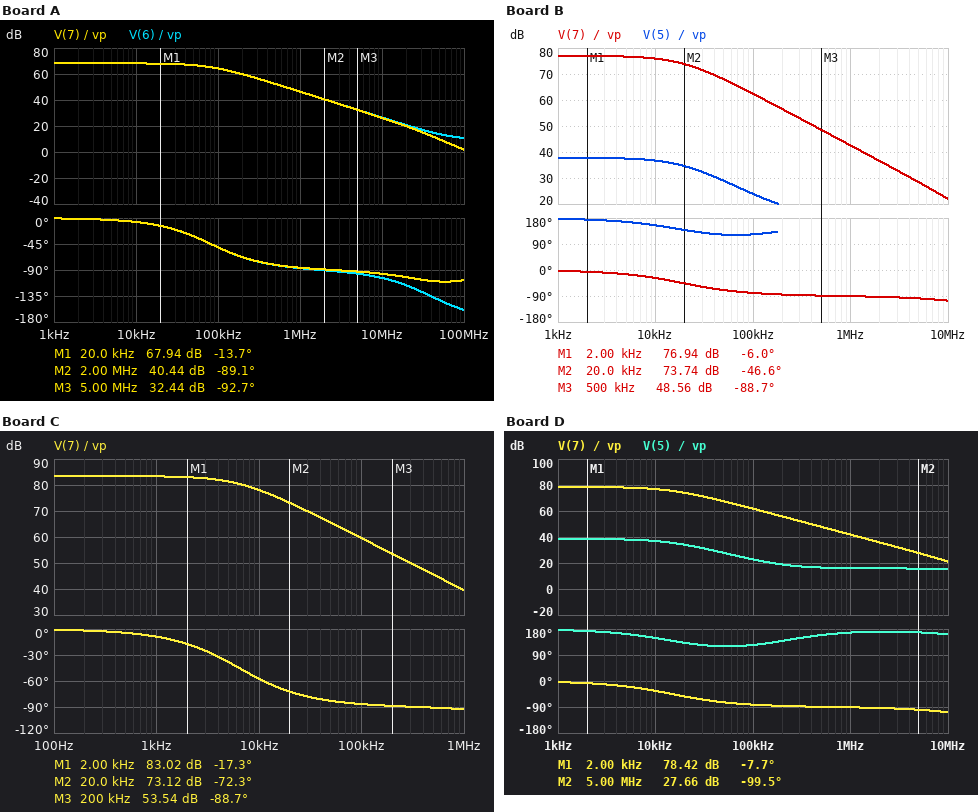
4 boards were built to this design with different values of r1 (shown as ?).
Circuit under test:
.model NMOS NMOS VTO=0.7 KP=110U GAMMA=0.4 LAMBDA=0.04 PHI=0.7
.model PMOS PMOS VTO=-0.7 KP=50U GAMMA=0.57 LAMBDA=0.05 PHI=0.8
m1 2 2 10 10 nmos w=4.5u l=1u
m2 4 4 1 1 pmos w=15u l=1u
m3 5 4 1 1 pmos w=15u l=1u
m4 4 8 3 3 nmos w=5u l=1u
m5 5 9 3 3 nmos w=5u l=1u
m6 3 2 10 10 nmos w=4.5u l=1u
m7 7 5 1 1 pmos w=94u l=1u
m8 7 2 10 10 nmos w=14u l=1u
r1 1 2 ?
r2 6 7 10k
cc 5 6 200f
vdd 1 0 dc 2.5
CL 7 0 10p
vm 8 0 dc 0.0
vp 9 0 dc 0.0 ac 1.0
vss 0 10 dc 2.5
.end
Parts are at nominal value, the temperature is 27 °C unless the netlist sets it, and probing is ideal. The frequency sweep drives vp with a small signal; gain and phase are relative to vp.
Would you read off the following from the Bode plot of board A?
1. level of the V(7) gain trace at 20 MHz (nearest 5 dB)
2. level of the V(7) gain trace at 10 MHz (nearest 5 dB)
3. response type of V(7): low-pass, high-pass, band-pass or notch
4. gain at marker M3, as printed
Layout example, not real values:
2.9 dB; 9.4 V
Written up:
20 dB; 25 dB; low-pass; 32.44 dB
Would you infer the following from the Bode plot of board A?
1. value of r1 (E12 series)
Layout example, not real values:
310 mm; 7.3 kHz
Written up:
22 kΩ
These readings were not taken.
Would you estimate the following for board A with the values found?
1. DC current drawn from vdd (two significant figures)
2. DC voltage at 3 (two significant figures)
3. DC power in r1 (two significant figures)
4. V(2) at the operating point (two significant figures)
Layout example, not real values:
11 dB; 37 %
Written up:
840 µA; -1.2 V; 560 µW; -1.0 V
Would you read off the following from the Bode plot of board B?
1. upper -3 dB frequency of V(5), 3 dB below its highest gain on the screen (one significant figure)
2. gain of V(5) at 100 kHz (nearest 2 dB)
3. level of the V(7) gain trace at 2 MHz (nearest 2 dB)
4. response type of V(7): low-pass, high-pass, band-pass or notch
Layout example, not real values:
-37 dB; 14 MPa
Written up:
20 kHz; 24 dB; 36 dB; low-pass
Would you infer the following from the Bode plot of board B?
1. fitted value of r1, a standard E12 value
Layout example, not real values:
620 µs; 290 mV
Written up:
68 kΩ
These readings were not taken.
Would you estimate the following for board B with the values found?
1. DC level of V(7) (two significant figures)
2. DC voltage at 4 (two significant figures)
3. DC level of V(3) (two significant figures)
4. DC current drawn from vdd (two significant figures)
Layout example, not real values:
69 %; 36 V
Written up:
500 mV; 1.5 V; -1.0 V; 300 µA
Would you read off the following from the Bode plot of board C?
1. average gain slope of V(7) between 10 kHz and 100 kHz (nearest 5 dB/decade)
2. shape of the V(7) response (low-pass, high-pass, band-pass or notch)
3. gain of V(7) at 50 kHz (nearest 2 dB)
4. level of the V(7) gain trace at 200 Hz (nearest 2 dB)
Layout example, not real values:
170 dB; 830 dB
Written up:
-20 dB/decade; low-pass; 66 dB; 84 dB
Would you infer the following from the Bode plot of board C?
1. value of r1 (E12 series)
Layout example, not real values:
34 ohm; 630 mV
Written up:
150 kΩ
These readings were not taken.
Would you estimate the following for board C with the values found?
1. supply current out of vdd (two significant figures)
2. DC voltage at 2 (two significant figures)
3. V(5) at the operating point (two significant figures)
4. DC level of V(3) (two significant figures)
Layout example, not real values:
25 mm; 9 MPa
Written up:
140 µA; -1.5 V; 1.6 V; -910 mV
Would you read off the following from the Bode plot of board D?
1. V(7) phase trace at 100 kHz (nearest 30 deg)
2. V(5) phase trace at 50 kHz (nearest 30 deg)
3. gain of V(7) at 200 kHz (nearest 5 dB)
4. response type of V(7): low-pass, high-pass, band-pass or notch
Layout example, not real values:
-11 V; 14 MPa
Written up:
-90 deg; 120 deg; 55 dB; low-pass
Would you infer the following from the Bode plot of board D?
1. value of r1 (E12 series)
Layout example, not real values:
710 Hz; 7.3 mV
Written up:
82 kΩ
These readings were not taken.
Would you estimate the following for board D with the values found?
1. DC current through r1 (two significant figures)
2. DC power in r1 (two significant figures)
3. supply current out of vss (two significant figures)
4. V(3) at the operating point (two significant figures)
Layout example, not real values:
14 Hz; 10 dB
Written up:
47 µA; 180 µW; 250 µA; -980 mV
